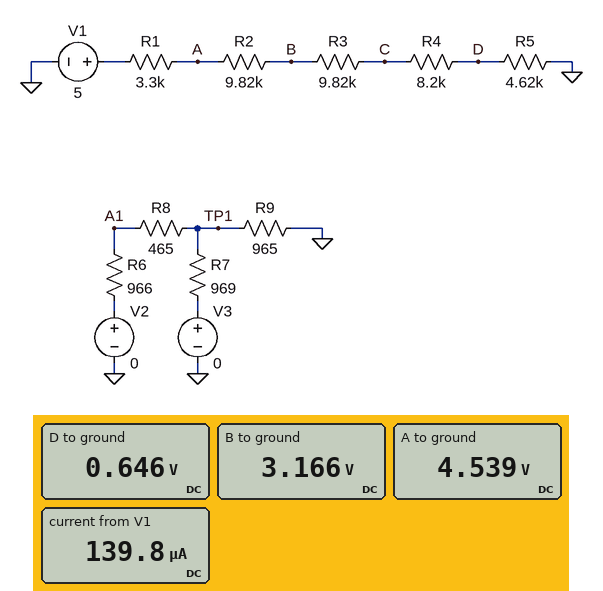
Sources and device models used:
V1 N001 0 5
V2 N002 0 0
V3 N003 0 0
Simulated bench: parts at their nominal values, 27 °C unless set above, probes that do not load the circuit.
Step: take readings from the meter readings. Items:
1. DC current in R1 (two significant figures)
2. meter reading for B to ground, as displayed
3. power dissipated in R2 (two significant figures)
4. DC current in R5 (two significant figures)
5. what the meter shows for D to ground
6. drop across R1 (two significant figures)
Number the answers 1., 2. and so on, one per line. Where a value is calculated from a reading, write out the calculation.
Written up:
1. (5 V - 4.539 V) / 3.3 kΩ = 140 µA
2. 3.166 V
3. (4.539 V - 3.166 V)^2 / 9.82 kΩ = 190 µW
4. (646 mV) / 4.62 kΩ = 140 µA
5. 0.646 V
6. 5 V - 4.539 V = 460 mV
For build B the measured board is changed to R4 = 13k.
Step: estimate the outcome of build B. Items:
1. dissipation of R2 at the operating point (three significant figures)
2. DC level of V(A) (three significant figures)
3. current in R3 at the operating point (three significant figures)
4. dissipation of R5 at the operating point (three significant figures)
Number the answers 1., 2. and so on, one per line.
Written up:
1. 149 µW
2. 4.59 V
3. 123 µA
4. 70.2 µW
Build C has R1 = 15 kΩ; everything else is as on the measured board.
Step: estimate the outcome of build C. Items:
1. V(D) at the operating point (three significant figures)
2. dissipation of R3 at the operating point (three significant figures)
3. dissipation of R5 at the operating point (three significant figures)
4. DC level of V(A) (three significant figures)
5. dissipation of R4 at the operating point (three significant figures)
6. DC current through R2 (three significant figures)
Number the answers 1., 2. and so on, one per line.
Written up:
1. 487 mV
2. 109 µW
3. 51.3 µW
4. 3.42 V
5. 91.0 µW
6. 105 µA
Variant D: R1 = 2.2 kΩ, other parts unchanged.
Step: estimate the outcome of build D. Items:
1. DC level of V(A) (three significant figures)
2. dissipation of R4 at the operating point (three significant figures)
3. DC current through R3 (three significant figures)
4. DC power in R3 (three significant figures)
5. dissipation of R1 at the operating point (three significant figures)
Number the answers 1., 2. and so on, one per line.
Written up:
1. 4.68 V
2. 171 µW
3. 144 µA
4. 204 µW
5. 45.8 µW
